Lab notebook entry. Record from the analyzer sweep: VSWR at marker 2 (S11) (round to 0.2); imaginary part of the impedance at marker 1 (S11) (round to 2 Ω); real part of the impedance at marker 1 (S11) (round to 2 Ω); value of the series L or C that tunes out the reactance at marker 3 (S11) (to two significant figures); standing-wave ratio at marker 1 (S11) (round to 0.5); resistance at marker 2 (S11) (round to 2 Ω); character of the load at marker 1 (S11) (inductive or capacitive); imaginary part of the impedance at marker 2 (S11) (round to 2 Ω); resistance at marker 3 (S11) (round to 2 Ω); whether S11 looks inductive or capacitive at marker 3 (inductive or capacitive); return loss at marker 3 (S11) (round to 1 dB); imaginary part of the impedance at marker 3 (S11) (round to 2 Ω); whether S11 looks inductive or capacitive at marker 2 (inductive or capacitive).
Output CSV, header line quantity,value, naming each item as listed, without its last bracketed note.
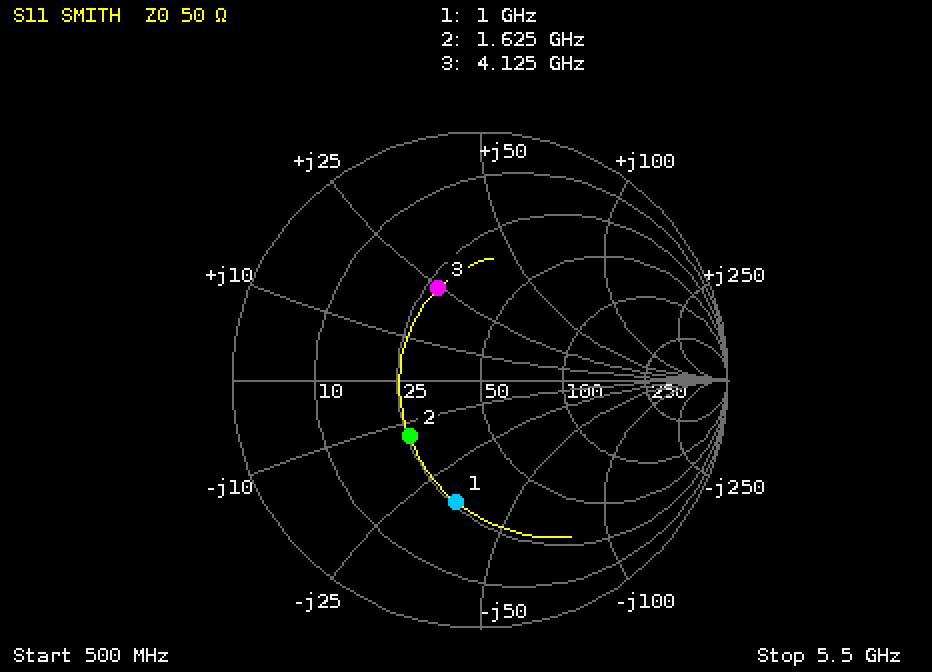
quantity,value
VSWR at marker 2 (S11),2.2
imaginary part of the impedance at marker 1 (S11),-34 Ω
real part of the impedance at marker 1 (S11),26 Ω
value of the series L or C that tunes out the reactance at marker 3 (S11),1.6 pF
standing-wave ratio at marker 1 (S11),3.0
resistance at marker 2 (S11),26 Ω
character of the load at marker 1 (S11),capacitive
imaginary part of the impedance at marker 2 (S11),-14 Ω
resistance at marker 3 (S11),28 Ω
whether S11 looks inductive or capacitive at marker 3,inductive
return loss at marker 3 (S11),8 dB
imaginary part of the impedance at marker 3 (S11),+24 Ω
whether S11 looks inductive or capacitive at marker 2,capacitive
